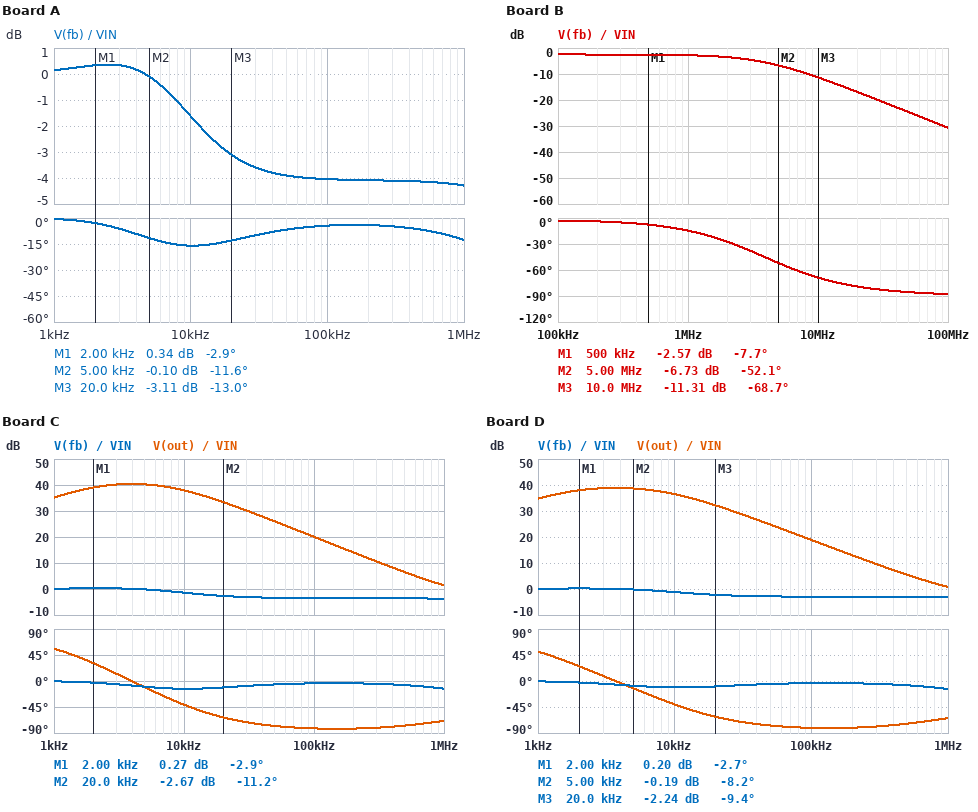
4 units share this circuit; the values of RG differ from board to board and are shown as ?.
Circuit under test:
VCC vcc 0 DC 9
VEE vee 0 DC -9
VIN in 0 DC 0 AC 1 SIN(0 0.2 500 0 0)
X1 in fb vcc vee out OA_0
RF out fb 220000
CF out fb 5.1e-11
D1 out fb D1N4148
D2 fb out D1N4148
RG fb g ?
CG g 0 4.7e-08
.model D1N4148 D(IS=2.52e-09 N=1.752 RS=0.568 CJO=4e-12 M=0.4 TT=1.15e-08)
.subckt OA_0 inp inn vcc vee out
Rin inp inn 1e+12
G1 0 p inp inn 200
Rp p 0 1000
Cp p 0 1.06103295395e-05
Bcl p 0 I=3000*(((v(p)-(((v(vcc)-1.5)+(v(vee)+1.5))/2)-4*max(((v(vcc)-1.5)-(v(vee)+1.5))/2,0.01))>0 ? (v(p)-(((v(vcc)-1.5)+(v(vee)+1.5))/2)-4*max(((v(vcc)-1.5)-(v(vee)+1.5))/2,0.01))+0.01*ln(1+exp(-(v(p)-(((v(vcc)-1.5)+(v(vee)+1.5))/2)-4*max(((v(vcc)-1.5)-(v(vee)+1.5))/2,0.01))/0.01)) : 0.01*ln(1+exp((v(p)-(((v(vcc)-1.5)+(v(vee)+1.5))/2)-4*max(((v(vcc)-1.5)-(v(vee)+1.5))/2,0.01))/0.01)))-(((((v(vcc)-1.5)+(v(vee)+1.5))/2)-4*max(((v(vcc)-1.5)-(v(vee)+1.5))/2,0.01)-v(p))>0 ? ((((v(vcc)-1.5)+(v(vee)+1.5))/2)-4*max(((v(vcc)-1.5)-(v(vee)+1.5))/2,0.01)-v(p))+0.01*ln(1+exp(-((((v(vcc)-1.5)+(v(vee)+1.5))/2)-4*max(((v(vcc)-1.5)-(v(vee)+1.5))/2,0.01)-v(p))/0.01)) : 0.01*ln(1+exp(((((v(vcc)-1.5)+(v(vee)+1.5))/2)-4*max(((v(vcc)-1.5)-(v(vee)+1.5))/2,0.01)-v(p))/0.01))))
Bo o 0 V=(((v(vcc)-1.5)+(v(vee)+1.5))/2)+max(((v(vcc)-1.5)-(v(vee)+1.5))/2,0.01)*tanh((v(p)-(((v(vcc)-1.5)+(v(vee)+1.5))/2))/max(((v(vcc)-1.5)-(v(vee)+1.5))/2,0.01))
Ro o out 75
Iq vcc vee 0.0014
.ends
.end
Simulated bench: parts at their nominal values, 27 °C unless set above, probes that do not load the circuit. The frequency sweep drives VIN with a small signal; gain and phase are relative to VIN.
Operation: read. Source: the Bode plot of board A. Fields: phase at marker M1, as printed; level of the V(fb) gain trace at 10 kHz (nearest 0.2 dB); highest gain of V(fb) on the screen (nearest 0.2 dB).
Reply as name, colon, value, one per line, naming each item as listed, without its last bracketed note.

phase at marker M1, as printed: -2.9 deg
level of the V(fb) gain trace at 10 kHz: -1.6 dB
highest gain of V(fb) on the screen: 0.4 dB
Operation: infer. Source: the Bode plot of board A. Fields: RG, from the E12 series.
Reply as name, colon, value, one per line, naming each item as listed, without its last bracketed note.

RG, from the E12 series: 1.5 kΩ
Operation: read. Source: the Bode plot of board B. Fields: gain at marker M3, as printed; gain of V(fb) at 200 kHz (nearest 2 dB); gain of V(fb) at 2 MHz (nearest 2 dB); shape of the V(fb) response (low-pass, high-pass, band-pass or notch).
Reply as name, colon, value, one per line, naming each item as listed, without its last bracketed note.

gain at marker M3, as printed: -11.31 dB
gain of V(fb) at 200 kHz: -2 dB
gain of V(fb) at 2 MHz: -4 dB
shape of the V(fb) response: low-pass
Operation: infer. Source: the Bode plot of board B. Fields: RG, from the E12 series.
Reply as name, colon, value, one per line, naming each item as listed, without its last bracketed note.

RG, from the E12 series: 2.7 kΩ
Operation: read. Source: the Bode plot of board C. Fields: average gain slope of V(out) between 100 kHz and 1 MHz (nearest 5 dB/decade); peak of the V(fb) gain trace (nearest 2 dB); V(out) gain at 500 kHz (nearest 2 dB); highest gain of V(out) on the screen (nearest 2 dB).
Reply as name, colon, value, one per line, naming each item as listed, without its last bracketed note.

average gain slope of V(out) between 100 kHz and 1 MHz: -20 dB/decade
peak of the V(fb) gain trace: 0 dB
V(out) gain at 500 kHz: 6 dB
highest gain of V(out) on the screen: 40 dB
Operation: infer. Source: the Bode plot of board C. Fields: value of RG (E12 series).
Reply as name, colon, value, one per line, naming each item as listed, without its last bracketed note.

value of RG: 1.8 kΩ
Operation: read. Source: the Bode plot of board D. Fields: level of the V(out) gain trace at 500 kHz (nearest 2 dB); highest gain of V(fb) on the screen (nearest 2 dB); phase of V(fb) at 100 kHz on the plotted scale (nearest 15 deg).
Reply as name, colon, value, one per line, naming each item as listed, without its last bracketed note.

level of the V(out) gain trace at 500 kHz: 6 dB
highest gain of V(fb) on the screen: 0 dB
phase of V(fb) at 100 kHz on the plotted scale: 0 deg
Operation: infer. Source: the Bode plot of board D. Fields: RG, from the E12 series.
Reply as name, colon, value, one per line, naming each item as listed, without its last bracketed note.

RG, from the E12 series: 2.2 kΩ
